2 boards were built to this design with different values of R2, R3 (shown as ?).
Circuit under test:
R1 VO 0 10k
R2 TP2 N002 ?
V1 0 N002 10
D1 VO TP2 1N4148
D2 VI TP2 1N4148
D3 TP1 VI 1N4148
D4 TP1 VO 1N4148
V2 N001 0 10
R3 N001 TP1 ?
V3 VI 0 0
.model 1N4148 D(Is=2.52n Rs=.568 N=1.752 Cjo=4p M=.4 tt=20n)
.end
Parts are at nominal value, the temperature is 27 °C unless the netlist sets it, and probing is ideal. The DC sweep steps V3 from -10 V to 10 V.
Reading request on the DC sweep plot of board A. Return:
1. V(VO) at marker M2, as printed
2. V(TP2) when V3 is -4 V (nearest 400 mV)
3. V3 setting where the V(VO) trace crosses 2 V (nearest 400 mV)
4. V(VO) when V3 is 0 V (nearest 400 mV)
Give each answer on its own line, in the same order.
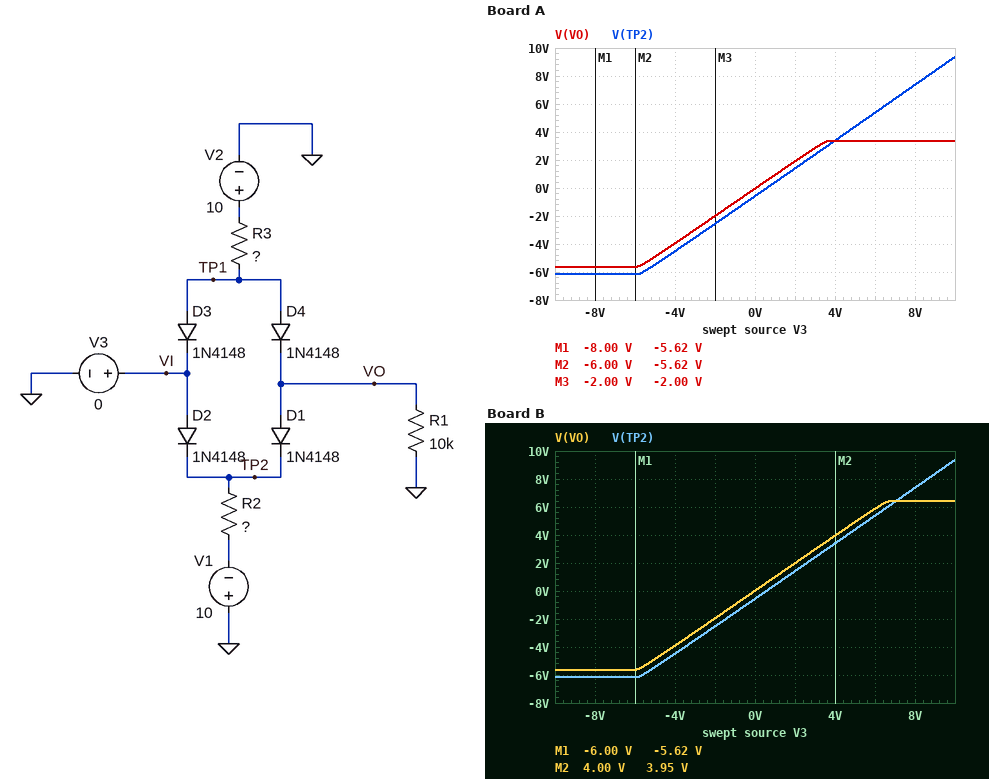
-5.62 V
-4.4 V
2.0 V
0 V
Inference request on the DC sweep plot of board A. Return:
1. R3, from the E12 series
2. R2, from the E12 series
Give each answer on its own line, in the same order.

18 kΩ
6.8 kΩ
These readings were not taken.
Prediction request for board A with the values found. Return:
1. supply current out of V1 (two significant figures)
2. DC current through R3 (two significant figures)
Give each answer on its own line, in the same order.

1.4 mA
530 µA
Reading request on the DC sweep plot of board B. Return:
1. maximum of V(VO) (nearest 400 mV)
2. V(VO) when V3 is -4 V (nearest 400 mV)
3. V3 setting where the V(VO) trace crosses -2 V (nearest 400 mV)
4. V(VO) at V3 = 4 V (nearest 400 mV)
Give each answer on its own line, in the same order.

6.4 V
-4.0 V
-2.0 V
4.0 V
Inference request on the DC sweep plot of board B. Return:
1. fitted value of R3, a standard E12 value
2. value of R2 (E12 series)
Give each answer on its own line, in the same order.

4.7 kΩ
6.8 kΩ
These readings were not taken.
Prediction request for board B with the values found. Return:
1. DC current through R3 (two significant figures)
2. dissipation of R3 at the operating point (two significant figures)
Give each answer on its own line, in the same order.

2.0 mA
19 mW
